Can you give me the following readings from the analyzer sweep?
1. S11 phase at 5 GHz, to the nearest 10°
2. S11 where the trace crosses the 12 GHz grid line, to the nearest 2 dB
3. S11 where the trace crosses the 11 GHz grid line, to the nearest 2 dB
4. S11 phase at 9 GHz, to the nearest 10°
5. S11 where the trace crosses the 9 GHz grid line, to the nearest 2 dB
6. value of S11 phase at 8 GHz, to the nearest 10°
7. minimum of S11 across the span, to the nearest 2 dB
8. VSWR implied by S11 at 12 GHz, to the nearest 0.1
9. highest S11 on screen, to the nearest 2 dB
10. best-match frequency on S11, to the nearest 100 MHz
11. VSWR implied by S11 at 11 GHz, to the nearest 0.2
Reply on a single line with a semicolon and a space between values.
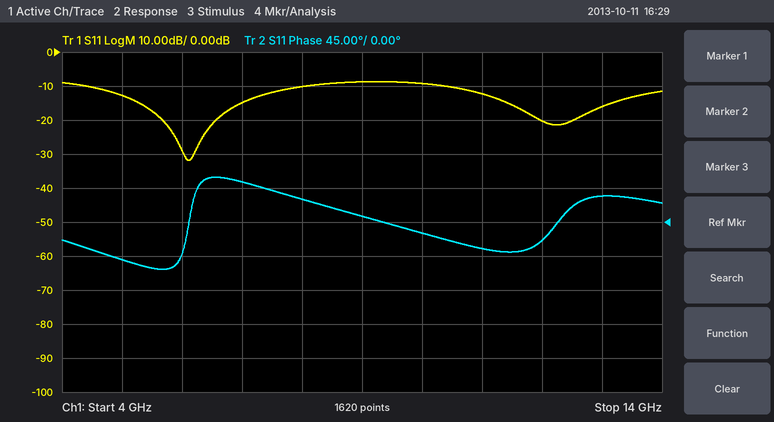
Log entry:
-50°; -20 dB; -12 dB; 10°; -8 dB; 30°; -32 dB; 1.2; -8 dB; 6.1 GHz; 1.6
